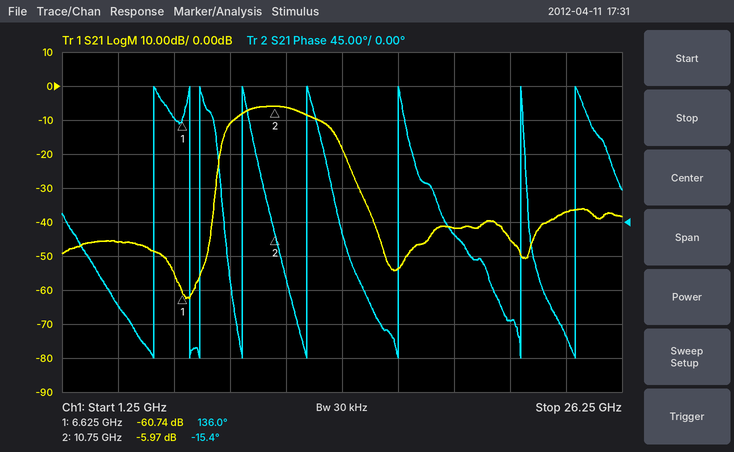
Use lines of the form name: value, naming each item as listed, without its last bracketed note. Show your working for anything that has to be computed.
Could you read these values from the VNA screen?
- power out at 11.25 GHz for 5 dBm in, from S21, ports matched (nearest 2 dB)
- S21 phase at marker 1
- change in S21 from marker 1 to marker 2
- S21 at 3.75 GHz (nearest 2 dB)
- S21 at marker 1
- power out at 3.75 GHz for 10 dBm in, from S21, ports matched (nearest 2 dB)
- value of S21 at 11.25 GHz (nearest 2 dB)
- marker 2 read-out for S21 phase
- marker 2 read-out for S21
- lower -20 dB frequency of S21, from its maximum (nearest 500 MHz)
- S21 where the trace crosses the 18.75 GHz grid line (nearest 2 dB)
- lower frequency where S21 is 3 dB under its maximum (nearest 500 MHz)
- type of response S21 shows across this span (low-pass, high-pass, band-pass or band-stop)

power out at 11.25 GHz for 5 dBm in, from S21, ports matched: 5 dBm + (-6 dB) = -2 dBm
S21 phase at marker 1: 136.0°
change in S21 from marker 1 to marker 2: -5.97 − (-60.74) = 54.77 dB
S21 at 3.75 GHz: -46 dB
S21 at marker 1: -60.74 dB
power out at 3.75 GHz for 10 dBm in, from S21, ports matched: 10 dBm + (-46 dB) = -36 dBm
value of S21 at 11.25 GHz: -6 dB
marker 2 read-out for S21 phase: -15.4°
marker 2 read-out for S21: -5.97 dB
lower -20 dB frequency of S21, from its maximum: 8.0 GHz
S21 where the trace crosses the 18.75 GHz grid line: -42 dB
lower frequency where S21 is 3 dB under its maximum: 9.0 GHz
type of response S21 shows across this span: band-pass
